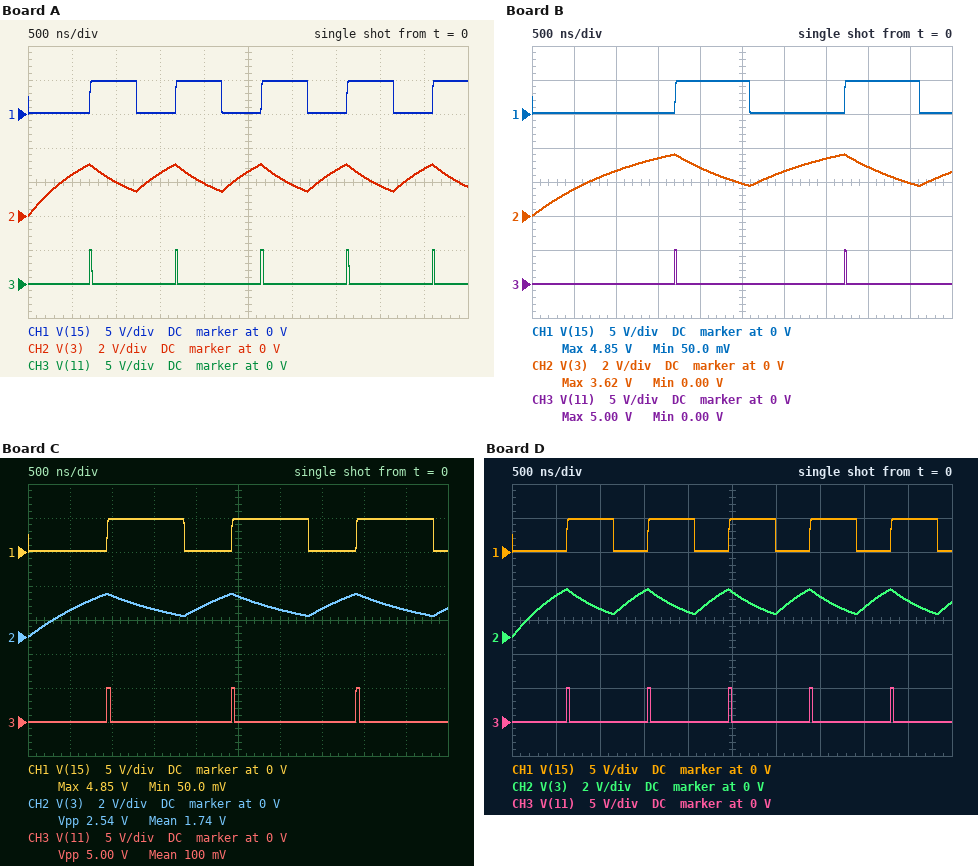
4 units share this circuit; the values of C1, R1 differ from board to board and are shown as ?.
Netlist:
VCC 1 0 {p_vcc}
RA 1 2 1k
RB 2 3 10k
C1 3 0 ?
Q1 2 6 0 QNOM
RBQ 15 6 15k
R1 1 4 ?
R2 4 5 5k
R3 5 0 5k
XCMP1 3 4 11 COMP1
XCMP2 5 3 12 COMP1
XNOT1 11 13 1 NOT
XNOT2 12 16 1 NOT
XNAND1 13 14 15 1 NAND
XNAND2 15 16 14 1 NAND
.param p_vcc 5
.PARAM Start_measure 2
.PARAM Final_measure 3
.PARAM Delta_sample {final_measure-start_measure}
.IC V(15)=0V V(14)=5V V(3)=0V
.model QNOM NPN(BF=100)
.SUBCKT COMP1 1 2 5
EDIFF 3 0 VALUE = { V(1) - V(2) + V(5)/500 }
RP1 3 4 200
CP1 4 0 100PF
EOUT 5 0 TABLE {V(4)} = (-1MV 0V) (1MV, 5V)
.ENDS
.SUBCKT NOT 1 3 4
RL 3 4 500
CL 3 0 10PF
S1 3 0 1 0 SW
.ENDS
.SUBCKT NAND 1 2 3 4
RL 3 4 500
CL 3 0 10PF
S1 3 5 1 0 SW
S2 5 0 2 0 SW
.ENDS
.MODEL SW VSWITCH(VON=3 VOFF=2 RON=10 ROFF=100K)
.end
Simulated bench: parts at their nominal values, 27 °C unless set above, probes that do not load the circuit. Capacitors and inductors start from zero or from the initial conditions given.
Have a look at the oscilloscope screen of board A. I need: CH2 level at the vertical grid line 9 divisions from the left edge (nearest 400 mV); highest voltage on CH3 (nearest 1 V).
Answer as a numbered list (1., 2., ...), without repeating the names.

1. 2.8 V
2. 5 V
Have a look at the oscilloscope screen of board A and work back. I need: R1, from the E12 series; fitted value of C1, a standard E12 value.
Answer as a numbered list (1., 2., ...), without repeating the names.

1. 6.8 kΩ
2. 68 pF
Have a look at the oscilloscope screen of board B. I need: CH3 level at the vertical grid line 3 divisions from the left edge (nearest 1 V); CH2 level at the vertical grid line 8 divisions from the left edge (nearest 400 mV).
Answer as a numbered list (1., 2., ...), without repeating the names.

1. 0 V
2. 2.8 V
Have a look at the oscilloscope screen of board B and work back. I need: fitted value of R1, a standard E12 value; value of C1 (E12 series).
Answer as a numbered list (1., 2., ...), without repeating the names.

1. 3.9 kΩ
2. 120 pF
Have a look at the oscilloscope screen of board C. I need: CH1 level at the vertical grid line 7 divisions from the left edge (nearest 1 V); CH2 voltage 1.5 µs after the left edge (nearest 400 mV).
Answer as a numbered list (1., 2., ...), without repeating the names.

1. 0 V
2. 1.6 V
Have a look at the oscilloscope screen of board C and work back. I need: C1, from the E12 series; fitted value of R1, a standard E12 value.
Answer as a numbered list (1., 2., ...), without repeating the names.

1. 120 pF
2. 10 kΩ
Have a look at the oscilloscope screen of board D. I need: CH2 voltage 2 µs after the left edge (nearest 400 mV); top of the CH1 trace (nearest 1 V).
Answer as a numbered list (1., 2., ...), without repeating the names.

1. 1.6 V
2. 5 V
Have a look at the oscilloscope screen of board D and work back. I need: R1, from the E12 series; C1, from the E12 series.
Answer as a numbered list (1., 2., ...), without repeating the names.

1. 8.2 kΩ
2. 68 pF
